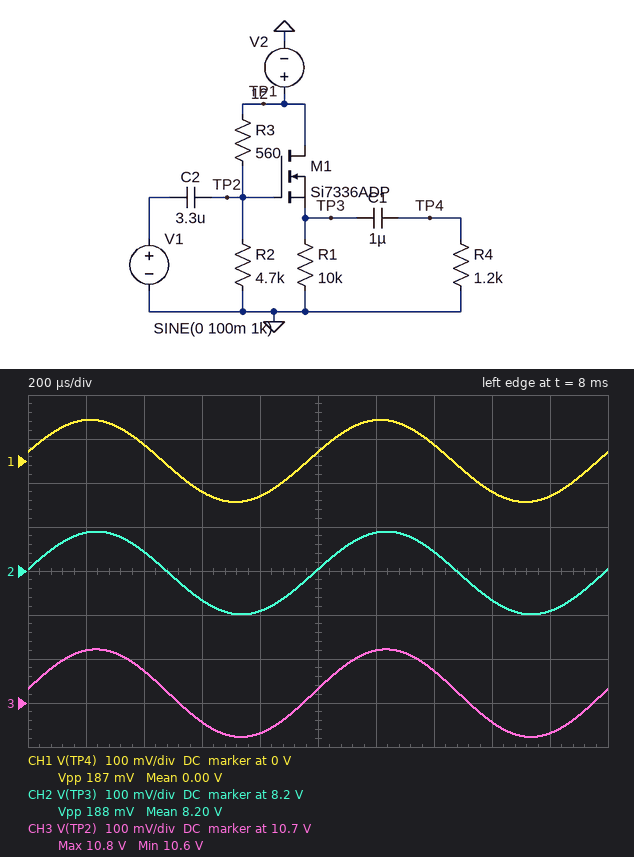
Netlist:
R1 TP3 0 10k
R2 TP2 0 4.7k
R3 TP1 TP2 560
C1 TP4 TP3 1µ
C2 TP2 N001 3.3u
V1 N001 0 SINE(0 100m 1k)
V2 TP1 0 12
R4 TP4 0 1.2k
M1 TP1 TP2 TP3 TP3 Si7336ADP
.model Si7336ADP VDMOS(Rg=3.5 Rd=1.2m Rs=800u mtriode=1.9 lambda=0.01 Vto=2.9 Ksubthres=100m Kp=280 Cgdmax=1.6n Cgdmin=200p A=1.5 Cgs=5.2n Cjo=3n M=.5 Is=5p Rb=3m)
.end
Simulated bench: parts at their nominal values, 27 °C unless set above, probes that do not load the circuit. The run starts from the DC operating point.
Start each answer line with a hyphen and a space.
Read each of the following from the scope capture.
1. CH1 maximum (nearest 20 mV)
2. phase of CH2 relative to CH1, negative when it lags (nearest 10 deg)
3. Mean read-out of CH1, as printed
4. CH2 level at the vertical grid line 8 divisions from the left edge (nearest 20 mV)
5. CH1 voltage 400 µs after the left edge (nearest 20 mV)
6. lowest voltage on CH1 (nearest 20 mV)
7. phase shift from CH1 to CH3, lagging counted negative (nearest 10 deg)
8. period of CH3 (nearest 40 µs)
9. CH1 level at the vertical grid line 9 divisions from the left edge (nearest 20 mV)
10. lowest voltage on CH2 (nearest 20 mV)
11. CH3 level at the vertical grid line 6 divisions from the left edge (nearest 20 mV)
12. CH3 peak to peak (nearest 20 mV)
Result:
- 100 mV
- -10 deg
- 0.00 V
- 8.14 V
- 40 mV
- -100 mV
- -10 deg
- 1.00 ms
- -80 mV
- 8.10 V
- 10.82 V
- 200 mV
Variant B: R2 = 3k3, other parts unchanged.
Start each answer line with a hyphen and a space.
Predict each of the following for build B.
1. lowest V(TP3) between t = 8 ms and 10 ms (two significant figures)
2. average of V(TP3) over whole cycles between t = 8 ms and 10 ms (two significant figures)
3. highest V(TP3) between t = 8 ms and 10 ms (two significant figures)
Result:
- 7.6 V
- 7.7 V
- 7.8 V
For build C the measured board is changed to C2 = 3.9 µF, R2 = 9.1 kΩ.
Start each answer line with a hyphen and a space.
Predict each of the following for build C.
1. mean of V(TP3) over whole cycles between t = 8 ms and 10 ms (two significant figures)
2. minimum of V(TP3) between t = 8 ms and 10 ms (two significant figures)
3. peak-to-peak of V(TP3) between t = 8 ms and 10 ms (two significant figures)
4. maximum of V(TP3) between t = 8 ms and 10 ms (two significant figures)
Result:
- 8.8 V
- 8.7 V
- 190 mV
- 8.9 V
